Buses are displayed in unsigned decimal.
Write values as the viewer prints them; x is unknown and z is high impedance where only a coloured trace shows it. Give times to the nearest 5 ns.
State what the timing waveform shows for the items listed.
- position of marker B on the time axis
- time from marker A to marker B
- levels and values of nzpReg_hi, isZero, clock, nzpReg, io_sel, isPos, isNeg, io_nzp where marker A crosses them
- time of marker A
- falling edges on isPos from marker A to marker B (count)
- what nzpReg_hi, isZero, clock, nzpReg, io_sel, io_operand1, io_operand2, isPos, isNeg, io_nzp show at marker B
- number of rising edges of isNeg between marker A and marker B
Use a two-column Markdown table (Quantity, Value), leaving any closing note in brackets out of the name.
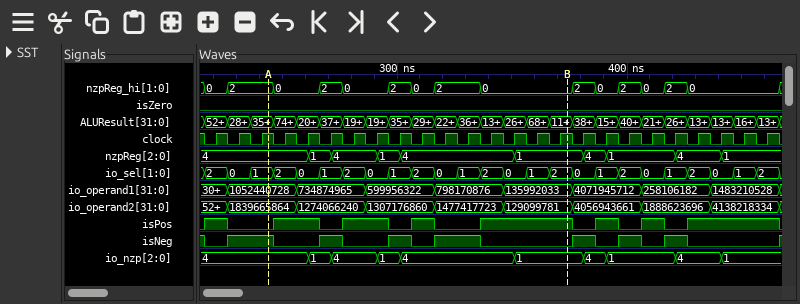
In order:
| Quantity | Value |
|---|---|
| position of marker B on the time axis | 375 ns |
| time from marker A to marker B | 130 ns |
| levels and values of nzpReg_hi, isZero, clock, nzpReg, io_sel, isPos, isNeg, io_nzp where marker A crosses them | nzpReg_hi=2, isZero=0, clock=1, nzpReg=4, io_sel=1, isPos=0, isNeg=1, io_nzp=4 |
| time of marker A | 245 ns |
| falling edges on isPos from marker A to marker B | 3 |
| what nzpReg_hi, isZero, clock, nzpReg, io_sel, io_operand1, io_operand2, isPos, isNeg, io_nzp show at marker B | nzpReg_hi=0, isZero=0, clock=1, nzpReg=1, io_sel=2, io_operand1=135992033, io_operand2=129099781, isPos=1, isNeg=0, io_nzp=1 |
| number of rising edges of isNeg between marker A and marker B | 3 |
